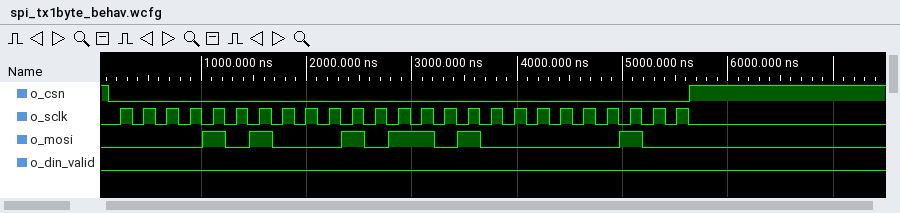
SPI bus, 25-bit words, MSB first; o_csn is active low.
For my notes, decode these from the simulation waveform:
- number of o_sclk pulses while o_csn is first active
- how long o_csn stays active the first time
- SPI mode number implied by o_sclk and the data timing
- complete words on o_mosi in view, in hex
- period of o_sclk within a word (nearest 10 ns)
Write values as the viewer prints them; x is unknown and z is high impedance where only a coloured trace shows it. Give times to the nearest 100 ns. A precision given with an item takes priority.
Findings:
25
5500 ns
0
0145A04
220 ns
